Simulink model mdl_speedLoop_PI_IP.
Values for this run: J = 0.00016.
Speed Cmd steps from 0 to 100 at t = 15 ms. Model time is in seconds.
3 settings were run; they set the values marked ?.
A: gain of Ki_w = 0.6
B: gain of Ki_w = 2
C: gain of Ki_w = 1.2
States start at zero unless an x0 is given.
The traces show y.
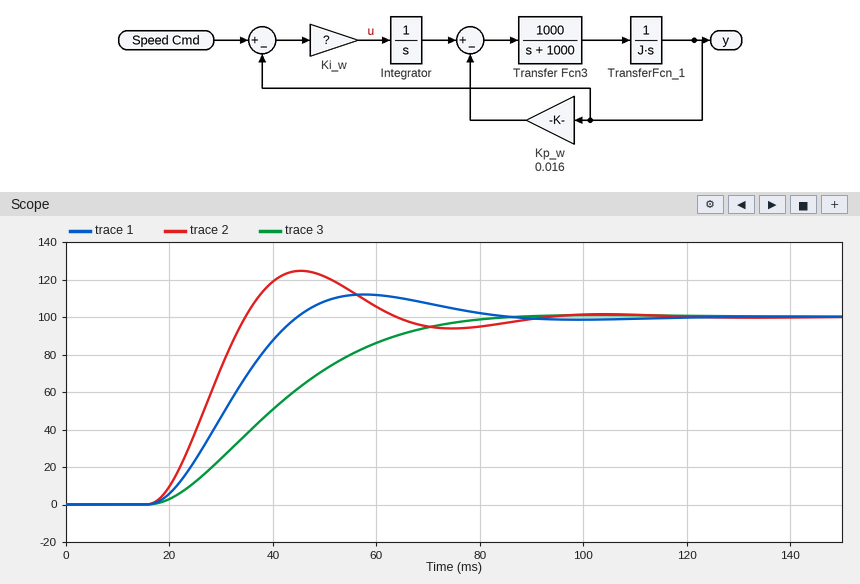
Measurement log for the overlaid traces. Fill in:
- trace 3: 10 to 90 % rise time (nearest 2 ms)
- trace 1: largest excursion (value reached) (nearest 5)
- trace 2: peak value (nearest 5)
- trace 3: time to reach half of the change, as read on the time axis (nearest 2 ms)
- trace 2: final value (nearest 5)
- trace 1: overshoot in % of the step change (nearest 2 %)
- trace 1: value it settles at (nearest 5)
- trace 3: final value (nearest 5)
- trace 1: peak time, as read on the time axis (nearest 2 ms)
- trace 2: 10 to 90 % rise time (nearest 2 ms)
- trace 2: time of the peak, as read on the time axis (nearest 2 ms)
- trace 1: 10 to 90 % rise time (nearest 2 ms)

40 ms
110
125
40 ms
100
12 %
100
100
58 ms
12 ms
46 ms
20 ms
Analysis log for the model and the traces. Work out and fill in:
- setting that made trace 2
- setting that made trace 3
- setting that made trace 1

B
A
C
